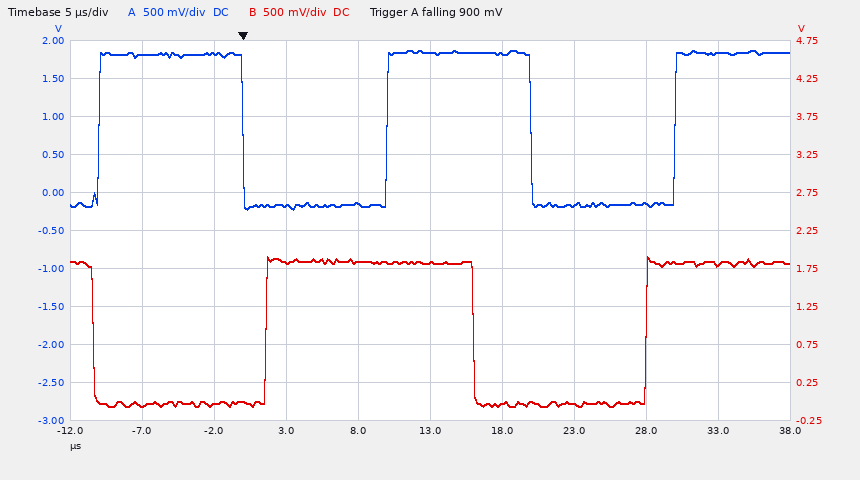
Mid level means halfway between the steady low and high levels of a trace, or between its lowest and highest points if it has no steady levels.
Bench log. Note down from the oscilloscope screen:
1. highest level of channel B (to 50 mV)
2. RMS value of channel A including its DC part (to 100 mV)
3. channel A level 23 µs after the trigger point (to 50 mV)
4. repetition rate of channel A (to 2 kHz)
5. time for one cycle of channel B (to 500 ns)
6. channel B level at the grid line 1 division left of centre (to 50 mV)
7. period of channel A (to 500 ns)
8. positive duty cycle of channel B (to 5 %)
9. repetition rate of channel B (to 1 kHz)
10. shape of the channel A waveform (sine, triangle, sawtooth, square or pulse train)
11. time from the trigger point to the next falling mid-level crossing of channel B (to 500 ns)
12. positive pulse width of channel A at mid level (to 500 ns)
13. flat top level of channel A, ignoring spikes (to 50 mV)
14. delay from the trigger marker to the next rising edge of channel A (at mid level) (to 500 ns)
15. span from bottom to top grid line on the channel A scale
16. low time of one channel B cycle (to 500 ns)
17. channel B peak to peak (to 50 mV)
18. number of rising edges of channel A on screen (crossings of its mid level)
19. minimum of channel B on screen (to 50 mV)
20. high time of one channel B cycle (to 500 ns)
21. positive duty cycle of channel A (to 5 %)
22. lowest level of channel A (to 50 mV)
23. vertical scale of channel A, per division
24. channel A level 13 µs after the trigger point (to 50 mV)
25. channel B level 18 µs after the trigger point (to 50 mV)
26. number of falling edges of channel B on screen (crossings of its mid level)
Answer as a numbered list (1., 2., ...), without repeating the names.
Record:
1. 1.90 V
2. 1.3 V
3. -150 mV
4. 50 kHz
5. 26.5 µs
6. 1.85 V
7. 20.0 µs
8. 55 %
9. 38 kHz
10. square
11. 16.0 µs
12. 10.0 µs
13. 1.85 V
14. 10.0 µs
15. 5 V
16. 12.0 µs
17. 1.95 V
18. 3
19. -50 mV
20. 14.5 µs
21. 50 %
22. -200 mV
23. 500 mV
24. 1.85 V
25. -50 mV
26. 2
